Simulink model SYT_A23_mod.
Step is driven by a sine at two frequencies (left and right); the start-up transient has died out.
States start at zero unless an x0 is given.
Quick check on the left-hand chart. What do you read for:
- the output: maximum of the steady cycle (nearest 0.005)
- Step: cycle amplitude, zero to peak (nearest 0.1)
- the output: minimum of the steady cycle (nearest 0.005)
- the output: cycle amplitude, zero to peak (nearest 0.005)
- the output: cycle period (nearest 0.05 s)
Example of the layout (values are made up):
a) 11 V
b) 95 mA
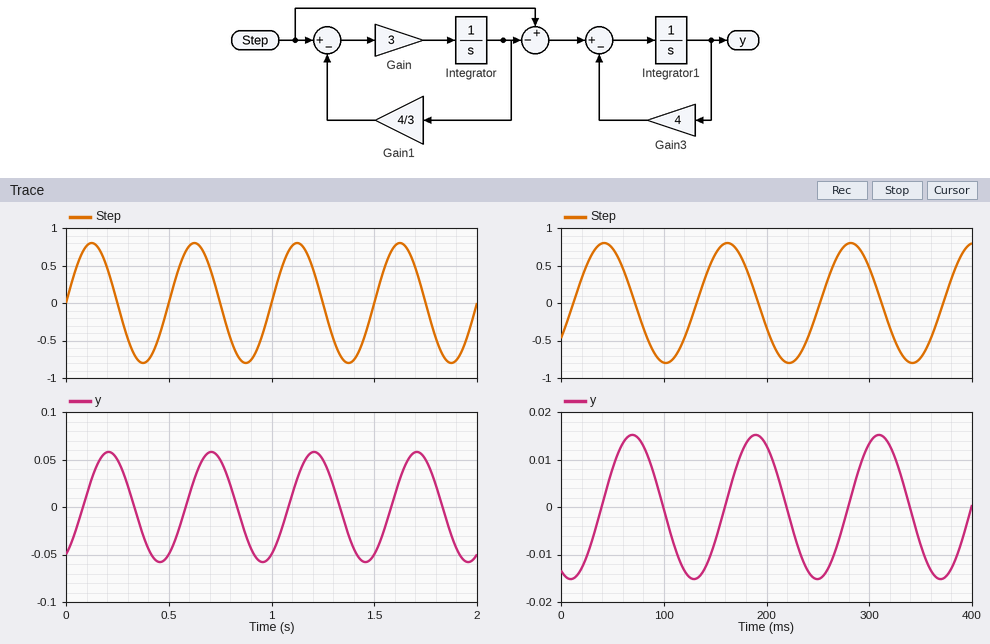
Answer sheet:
a) 0.060
b) 0.8
c) -0.060
d) 0.060
e) 0.50 s
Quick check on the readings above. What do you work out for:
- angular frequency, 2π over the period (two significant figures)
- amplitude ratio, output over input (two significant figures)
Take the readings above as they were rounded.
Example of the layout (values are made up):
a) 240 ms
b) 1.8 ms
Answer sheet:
a) 13 rad/s
b) 0.075
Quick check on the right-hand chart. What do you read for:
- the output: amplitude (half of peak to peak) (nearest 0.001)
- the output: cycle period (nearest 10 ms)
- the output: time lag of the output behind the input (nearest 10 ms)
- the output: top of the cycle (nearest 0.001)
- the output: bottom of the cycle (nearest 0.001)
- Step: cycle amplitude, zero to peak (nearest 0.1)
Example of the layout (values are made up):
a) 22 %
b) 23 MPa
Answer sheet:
a) 0.015
b) 120 ms
c) 30 ms
d) 0.015
e) -0.015
f) 0.8
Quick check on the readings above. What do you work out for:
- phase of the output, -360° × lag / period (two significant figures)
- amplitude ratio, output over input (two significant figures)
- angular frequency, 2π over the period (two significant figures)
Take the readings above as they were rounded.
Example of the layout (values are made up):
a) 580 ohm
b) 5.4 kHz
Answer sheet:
a) -90°
b) 0.019
c) 0.052 rad/ms
